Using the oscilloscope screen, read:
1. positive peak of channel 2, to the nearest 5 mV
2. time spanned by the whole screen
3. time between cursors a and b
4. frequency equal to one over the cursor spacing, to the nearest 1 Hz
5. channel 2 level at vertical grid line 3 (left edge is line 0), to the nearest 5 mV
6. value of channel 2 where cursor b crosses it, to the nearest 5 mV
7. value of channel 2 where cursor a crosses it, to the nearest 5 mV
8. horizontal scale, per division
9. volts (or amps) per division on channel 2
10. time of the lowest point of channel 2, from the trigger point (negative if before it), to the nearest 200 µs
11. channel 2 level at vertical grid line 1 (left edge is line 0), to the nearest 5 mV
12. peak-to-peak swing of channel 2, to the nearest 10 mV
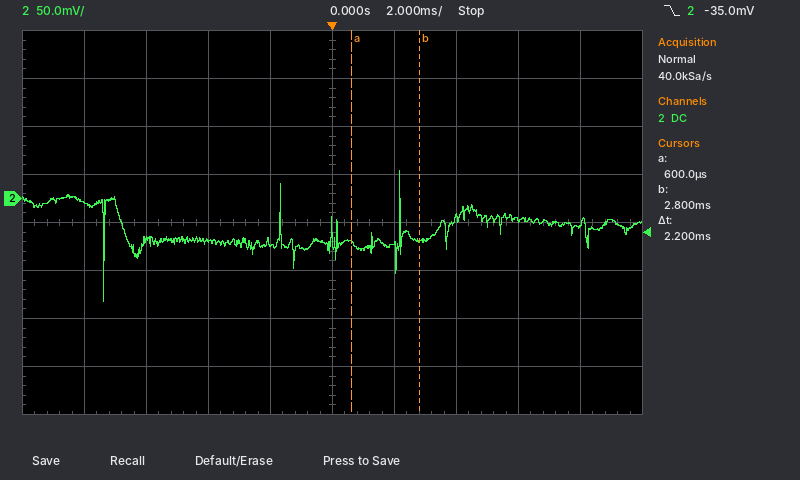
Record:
30 mV
20 ms
2.2 ms
455 Hz
-45 mV
-45 mV
-45 mV
2 ms
50 mV
-7.4 ms
-5 mV
140 mV
